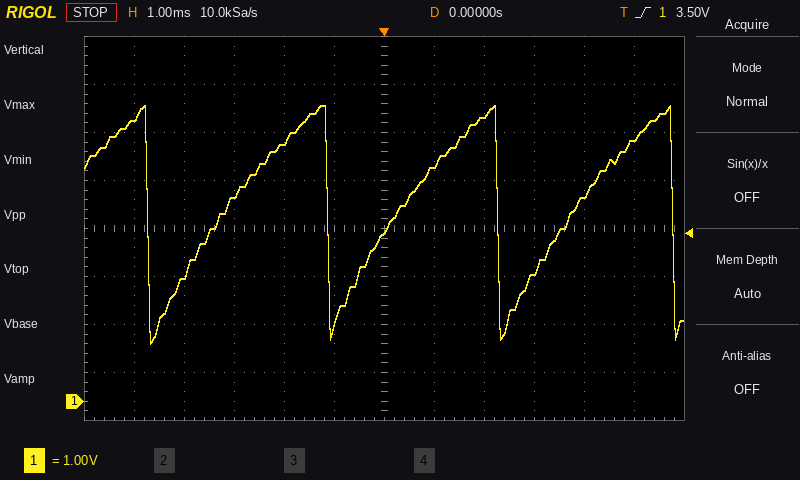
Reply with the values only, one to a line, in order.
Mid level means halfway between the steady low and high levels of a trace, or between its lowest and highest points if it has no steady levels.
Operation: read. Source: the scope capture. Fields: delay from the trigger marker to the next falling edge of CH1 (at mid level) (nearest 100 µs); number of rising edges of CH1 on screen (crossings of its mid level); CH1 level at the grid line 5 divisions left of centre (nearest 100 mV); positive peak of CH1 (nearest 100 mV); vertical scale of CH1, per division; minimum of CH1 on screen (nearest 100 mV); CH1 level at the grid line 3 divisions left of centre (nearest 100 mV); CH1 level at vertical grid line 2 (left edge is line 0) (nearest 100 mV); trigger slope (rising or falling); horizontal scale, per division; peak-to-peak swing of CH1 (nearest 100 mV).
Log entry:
2.3 ms
3
5.9 V
6.2 V
1 V
1.2 V
4.3 V
2.6 V
rising
1 ms
5.0 V
